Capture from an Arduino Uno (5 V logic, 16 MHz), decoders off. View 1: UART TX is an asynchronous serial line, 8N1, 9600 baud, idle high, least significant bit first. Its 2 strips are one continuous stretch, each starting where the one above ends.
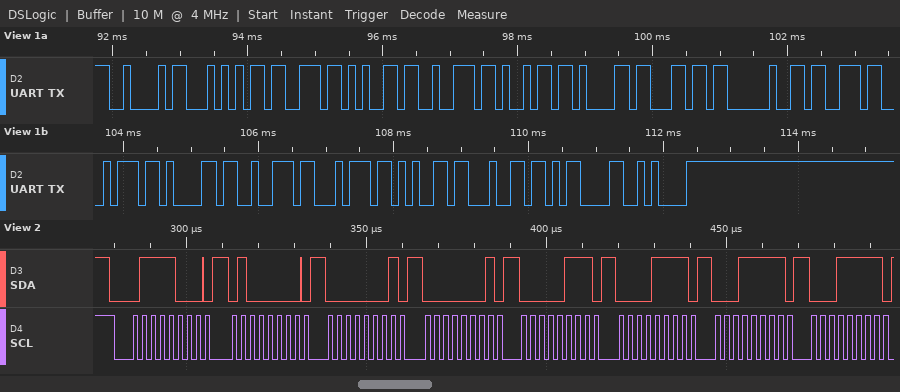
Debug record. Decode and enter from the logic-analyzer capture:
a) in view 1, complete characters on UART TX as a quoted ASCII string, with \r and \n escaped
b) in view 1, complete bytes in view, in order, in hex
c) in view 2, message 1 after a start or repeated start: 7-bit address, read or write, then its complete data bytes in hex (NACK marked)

"BTserial started\r\n"
42 54 73 65 72 69 61 6C 20 73 74 61 72 74 65 64 0D 0A
0x3C write: 40 01 01 07 0F 1F 1F
